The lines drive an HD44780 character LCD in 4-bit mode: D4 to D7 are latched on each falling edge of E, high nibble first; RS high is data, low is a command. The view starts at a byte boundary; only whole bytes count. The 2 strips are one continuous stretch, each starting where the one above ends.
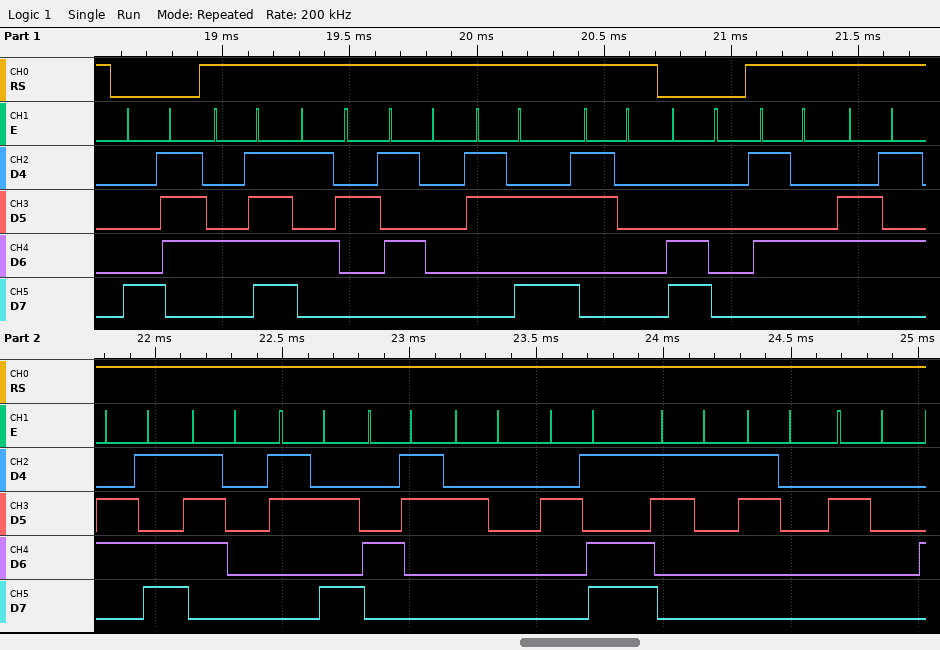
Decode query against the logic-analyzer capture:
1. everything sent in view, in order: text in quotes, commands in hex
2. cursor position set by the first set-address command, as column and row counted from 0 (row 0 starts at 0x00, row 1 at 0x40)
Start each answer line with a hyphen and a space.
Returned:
- 0x87 "ORP:0" 0xC0 "Temp:C -10 "
- column 7, row 0
